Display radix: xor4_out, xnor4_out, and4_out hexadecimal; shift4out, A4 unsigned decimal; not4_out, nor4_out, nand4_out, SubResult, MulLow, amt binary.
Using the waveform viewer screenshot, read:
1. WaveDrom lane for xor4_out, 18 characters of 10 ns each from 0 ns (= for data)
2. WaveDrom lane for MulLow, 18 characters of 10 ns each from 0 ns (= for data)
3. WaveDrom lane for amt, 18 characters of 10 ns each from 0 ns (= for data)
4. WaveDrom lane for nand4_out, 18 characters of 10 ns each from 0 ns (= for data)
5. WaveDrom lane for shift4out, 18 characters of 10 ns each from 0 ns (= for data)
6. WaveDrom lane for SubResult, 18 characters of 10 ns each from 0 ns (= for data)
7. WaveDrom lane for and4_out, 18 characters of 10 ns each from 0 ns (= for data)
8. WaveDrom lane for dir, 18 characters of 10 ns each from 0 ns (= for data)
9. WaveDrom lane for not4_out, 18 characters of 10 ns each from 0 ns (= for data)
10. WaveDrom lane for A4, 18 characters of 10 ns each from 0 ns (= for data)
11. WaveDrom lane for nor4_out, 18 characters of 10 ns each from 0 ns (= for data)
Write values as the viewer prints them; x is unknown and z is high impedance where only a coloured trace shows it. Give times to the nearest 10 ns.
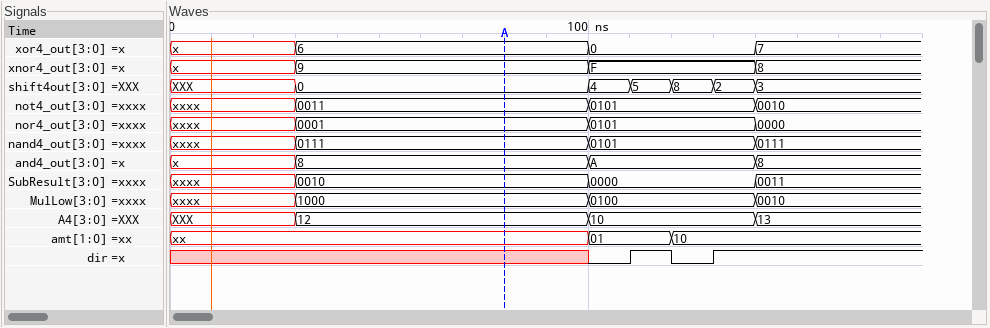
{name: 'xor4_out', wave: 'x..=......=...=...', data: '6 0 7'}
{name: 'MulLow', wave: 'x..=......=...=...', data: '1000 0100 0010'}
{name: 'amt', wave: 'x.........=.=.....', data: '01 10'}
{name: 'nand4_out', wave: 'x..=......=...=...', data: '0111 0101 0111'}
{name: 'shift4out', wave: 'x..=......=====...', data: '0 4 5 8 2 3'}
{name: 'SubResult', wave: 'x..=......=...=...', data: '0010 0000 0011'}
{name: 'and4_out', wave: 'x..=......=...=...', data: '8 A 8'}
{name: 'dir', wave: 'x.........0101....'}
{name: 'not4_out', wave: 'x..=......=...=...', data: '0011 0101 0010'}
{name: 'A4', wave: 'x..=......=...=...', data: '12 10 13'}
{name: 'nor4_out', wave: 'x..=......=...=...', data: '0001 0101 0000'}
